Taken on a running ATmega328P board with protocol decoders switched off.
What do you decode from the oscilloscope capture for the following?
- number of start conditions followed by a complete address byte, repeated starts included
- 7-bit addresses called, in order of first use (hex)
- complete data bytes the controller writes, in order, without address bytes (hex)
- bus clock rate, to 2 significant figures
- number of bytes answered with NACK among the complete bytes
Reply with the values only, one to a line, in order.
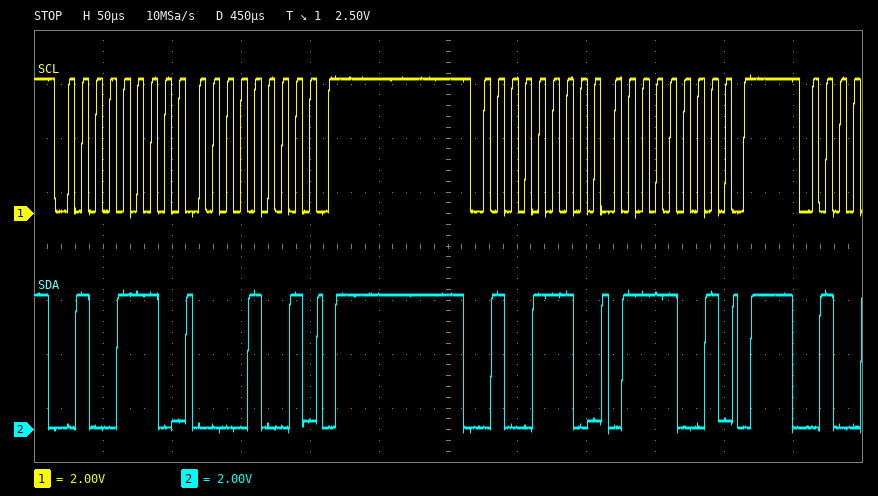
2
0x27
09 79
100 kHz
0
